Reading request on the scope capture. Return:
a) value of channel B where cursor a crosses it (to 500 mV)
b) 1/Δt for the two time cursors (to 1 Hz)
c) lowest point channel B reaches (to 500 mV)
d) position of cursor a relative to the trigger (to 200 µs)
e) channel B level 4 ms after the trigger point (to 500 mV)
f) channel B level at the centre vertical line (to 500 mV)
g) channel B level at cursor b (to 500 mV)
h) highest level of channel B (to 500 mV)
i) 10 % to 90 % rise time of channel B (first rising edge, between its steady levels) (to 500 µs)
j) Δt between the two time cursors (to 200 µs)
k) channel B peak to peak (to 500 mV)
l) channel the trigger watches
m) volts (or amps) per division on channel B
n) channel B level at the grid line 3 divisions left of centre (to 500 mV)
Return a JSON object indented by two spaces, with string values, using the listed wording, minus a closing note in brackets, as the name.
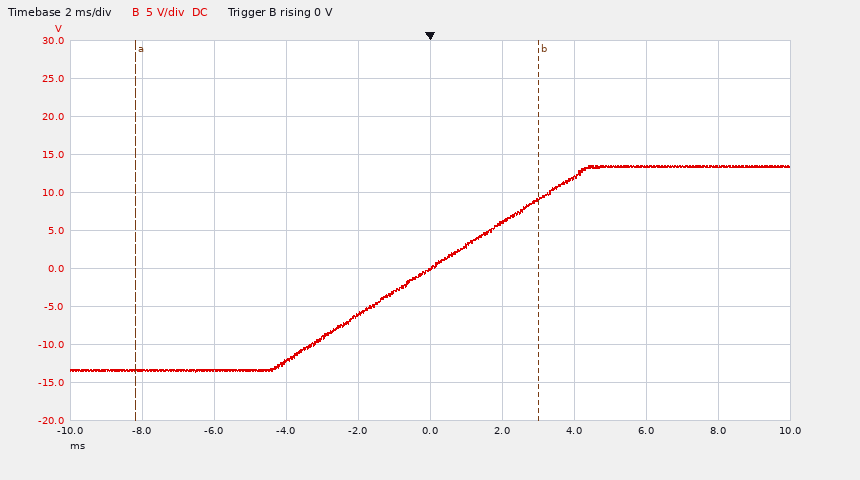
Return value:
{
  "value of channel B where cursor a crosses it": "-13.5 V",
  "1/Δt for the two time cursors": "89 Hz",
  "lowest point channel B reaches": "-13.5 V",
  "position of cursor a relative to the trigger": "-8.2 ms",
  "channel B level 4 ms after the trigger point": "12.0 V",
  "channel B level at the centre vertical line": "0.0 V",
  "channel B level at cursor b": "9.0 V",
  "highest level of channel B": "13.5 V",
  "10 % to 90 % rise time of channel B (first rising edge, between its steady levels)": "7.0 ms",
  "Δt between the two time cursors": "11.2 ms",
  "channel B peak to peak": "27.0 V",
  "channel the trigger watches": "channel B",
  "volts (or amps) per division on channel B": "5 V",
  "channel B level at the grid line 3 divisions left of centre": "-13.5 V"
}
